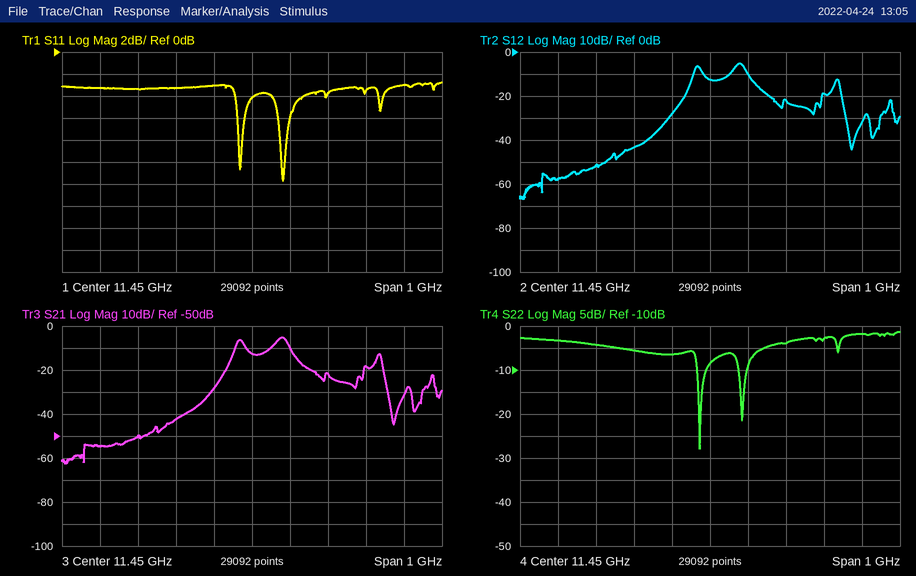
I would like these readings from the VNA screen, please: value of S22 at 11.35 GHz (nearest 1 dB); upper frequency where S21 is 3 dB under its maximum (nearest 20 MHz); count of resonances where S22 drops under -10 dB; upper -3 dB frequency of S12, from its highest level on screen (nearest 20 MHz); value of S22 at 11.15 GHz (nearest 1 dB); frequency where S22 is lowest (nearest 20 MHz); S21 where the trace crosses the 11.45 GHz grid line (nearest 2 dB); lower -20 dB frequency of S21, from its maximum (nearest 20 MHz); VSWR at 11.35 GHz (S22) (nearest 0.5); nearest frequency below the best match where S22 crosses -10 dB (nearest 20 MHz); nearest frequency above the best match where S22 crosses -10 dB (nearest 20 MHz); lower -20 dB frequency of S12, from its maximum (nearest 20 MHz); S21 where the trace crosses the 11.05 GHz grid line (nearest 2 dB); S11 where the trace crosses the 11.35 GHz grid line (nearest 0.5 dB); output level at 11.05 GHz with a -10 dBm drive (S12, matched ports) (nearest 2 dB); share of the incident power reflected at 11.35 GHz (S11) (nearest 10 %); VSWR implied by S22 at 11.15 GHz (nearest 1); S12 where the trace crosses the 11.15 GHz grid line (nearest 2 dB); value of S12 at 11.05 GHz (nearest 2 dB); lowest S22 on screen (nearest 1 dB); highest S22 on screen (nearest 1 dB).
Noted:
-6 dB
11.54 GHz
2
11.54 GHz
-4 dB
11.42 GHz
-12 dB
11.36 GHz
3.0
11.42 GHz
11.44 GHz
11.36 GHz
-54 dB
-3.0 dB
-68 dBm
50 %
4
-52 dB
-58 dB
-28 dB
-1 dB
